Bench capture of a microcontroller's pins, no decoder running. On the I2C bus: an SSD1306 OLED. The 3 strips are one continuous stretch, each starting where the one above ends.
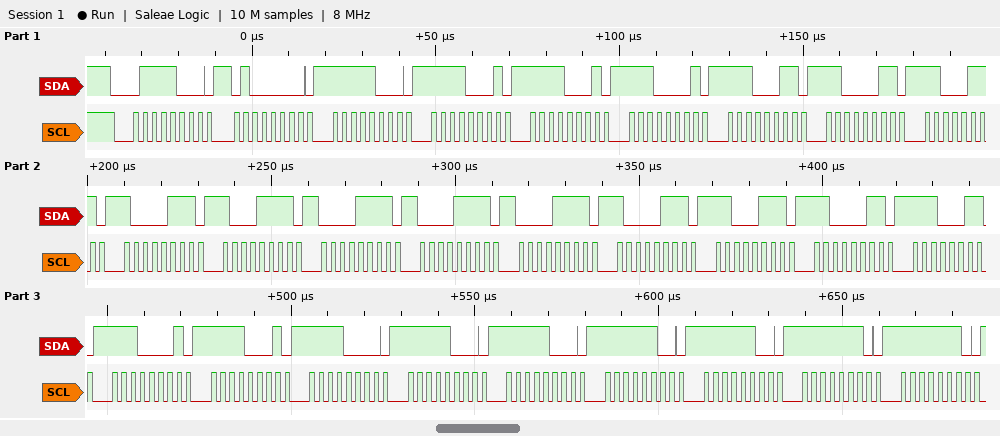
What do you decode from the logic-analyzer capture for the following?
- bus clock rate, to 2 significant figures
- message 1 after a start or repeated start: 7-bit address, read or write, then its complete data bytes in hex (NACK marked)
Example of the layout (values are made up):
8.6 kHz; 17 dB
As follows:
400 kHz; 0x3C write: 40 F8 F1 F1 E1 E3 C3 C7 87 8F 0F 0F 0F 87 C7 C3 E3 E1 F1 F0 F8 F8 FC FC FE FE
